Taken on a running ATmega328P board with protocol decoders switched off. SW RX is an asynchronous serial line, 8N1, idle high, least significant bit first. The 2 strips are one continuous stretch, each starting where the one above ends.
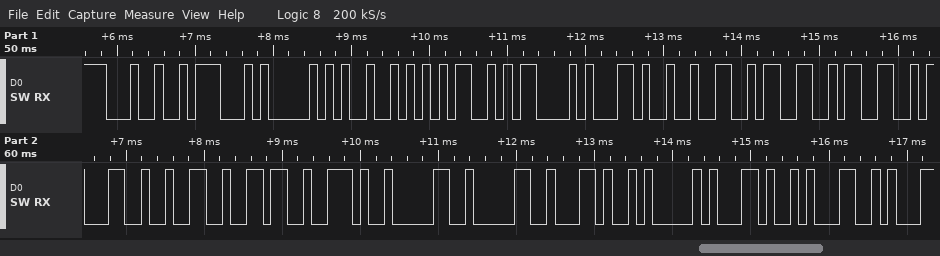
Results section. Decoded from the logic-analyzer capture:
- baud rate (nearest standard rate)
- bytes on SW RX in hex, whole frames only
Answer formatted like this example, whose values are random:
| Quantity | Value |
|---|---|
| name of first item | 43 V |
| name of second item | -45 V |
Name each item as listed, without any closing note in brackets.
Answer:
| Quantity | Value |
|---|---|
| baud rate | 9600 baud |
| bytes on SW RX in hex, whole frames only | 24 47 50 52 4D 43 2C 32 33 33 31 32 36 2E 30 30 2C 41 2C 31 |
